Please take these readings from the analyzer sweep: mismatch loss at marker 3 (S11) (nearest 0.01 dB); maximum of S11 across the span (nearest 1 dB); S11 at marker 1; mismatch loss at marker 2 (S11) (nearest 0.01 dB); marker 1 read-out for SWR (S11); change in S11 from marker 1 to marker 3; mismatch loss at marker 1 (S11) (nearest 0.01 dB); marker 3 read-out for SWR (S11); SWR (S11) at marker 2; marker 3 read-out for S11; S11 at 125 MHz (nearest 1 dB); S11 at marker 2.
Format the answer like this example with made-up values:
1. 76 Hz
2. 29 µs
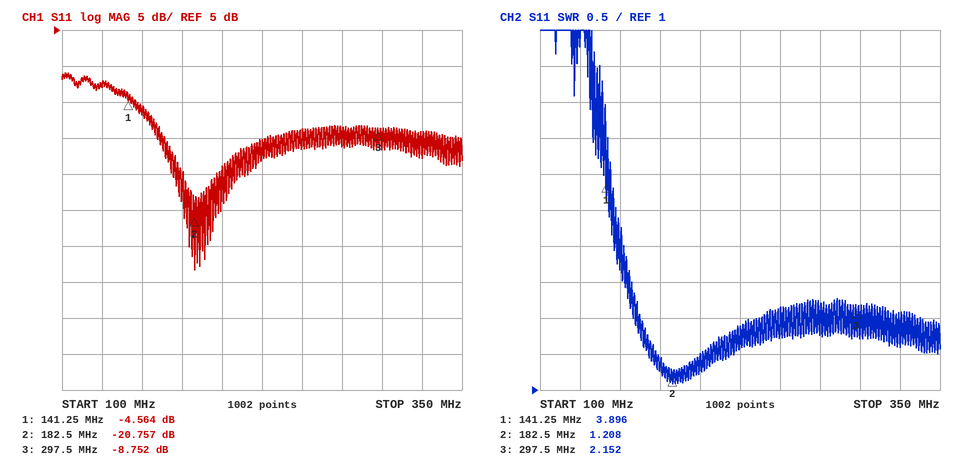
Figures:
1. 0.62 dB
2. -1 dB
3. -4.564 dB
4. 0.04 dB
5. 3.896
6. -4.188 dB
7. 1.87 dB
8. 2.152
9. 1.208
10. -8.752 dB
11. -3 dB
12. -20.757 dB
